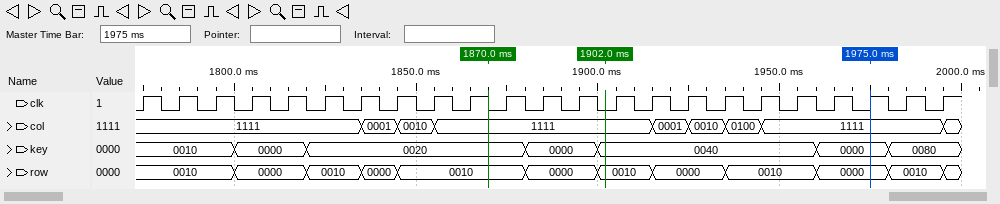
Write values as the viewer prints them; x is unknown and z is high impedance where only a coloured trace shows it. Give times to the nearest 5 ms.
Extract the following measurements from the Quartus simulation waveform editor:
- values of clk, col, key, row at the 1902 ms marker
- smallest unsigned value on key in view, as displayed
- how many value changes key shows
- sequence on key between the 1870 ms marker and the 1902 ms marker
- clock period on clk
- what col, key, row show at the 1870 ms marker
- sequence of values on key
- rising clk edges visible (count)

clk=0, col=1111, key=0040, row=0010
0000
6
0020, 0000, 0040
10 ms
col=1111, key=0020, row=0010
0010, 0000, 0020, 0000, 0040, 0000, 0080
23
